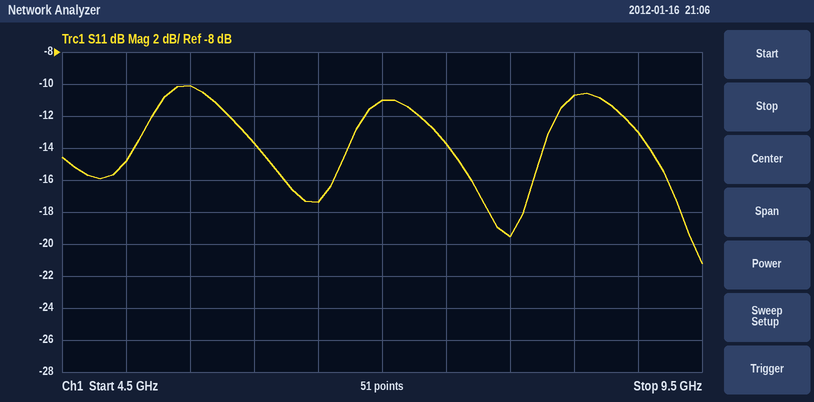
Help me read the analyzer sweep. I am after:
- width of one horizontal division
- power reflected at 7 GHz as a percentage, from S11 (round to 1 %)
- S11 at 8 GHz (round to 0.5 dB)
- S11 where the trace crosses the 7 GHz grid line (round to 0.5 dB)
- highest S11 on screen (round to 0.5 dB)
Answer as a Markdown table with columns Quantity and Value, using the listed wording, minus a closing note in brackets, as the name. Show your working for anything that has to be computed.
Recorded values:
| Quantity | Value |
|---|---|
| width of one horizontal division | 500 MHz |
| power reflected at 7 GHz as a percentage, from S11 | 10^(-11/10) ≈ 8 % |
| S11 at 8 GHz | -19.5 dB |
| S11 where the trace crosses the 7 GHz grid line | -11.0 dB |
| highest S11 on screen | -10.0 dB |
